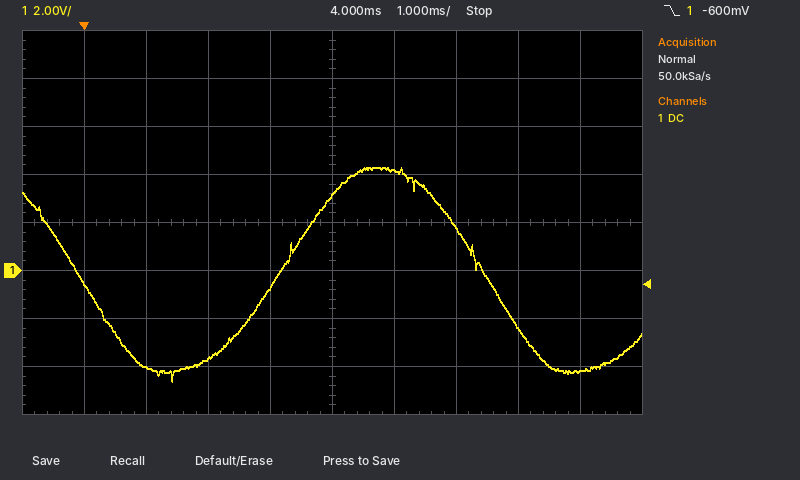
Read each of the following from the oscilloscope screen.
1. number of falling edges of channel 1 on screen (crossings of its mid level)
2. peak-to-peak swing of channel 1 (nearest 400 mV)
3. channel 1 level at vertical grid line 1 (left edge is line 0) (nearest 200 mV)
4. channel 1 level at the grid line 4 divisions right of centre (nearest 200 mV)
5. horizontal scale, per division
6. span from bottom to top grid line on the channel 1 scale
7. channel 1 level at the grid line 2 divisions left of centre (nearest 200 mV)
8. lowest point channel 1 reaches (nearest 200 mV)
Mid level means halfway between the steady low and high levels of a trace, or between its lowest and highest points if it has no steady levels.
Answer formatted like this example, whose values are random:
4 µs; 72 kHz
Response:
2; 8.8 V; -600 mV; -4.2 V; 1 ms; 16 V; -3.6 V; -4.6 V
